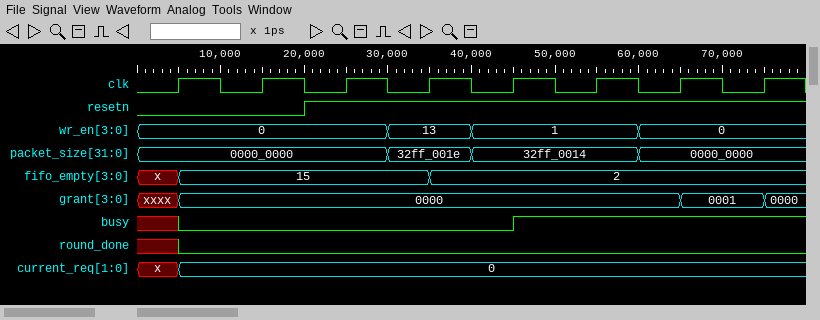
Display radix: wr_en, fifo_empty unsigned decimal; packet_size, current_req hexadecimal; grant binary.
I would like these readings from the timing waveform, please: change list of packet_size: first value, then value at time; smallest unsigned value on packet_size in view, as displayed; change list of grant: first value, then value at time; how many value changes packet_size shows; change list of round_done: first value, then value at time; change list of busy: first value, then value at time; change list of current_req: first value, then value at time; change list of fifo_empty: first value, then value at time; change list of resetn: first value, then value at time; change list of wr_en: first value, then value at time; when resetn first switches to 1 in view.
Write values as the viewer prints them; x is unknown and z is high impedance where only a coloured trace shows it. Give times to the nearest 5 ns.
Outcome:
0000_0000, 32ff_001e at 30 ns, 32ff_0014 at 40 ns, 0000_0000 at 60 ns
0000_0000
xxxx, 0000 at 5 ns, 0001 at 65 ns, 0000 at 75 ns
3
x, 0 at 5 ns
x, 0 at 5 ns, 1 at 45 ns
x, 0 at 5 ns
x, 15 at 5 ns, 2 at 35 ns
0, 1 at 20 ns
0, 13 at 30 ns, 1 at 40 ns, 0 at 60 ns
20 ns
